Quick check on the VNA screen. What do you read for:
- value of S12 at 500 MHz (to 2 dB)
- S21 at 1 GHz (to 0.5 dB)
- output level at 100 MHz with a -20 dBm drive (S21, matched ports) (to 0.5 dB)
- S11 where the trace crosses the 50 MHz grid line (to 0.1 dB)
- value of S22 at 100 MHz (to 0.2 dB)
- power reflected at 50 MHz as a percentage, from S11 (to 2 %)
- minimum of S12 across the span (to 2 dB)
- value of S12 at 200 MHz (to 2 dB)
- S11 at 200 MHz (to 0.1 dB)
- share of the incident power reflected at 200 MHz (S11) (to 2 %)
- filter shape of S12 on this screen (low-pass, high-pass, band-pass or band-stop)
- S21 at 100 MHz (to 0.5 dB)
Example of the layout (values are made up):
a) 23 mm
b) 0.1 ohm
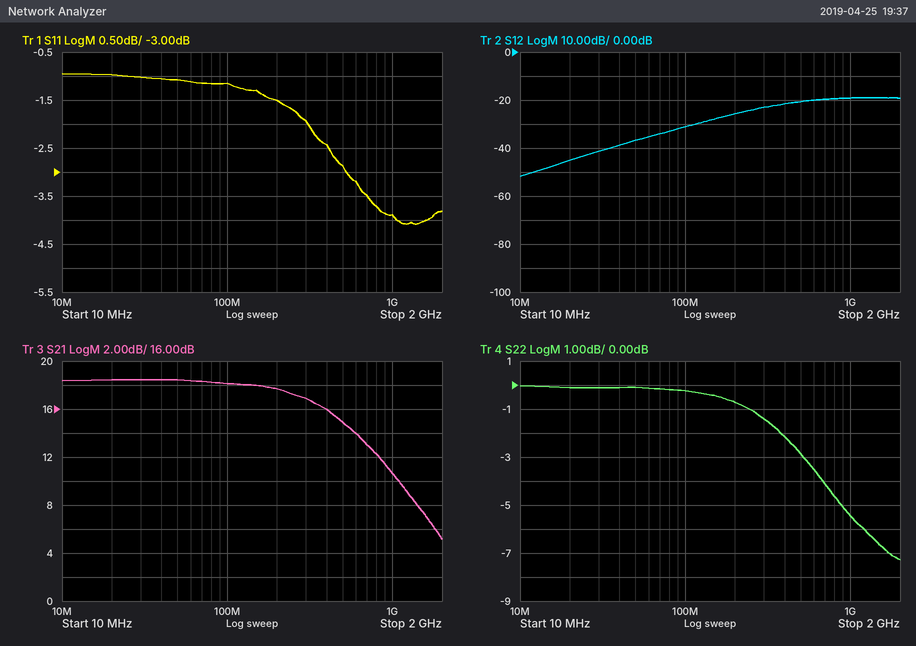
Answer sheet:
a) -20 dB
b) 10.5 dB
c) -2.0 dBm
d) -1.1 dB
e) -0.2 dB
f) 78 %
g) -52 dB
h) -26 dB
i) -1.5 dB
j) 70 %
k) high-pass
l) 18.0 dB
